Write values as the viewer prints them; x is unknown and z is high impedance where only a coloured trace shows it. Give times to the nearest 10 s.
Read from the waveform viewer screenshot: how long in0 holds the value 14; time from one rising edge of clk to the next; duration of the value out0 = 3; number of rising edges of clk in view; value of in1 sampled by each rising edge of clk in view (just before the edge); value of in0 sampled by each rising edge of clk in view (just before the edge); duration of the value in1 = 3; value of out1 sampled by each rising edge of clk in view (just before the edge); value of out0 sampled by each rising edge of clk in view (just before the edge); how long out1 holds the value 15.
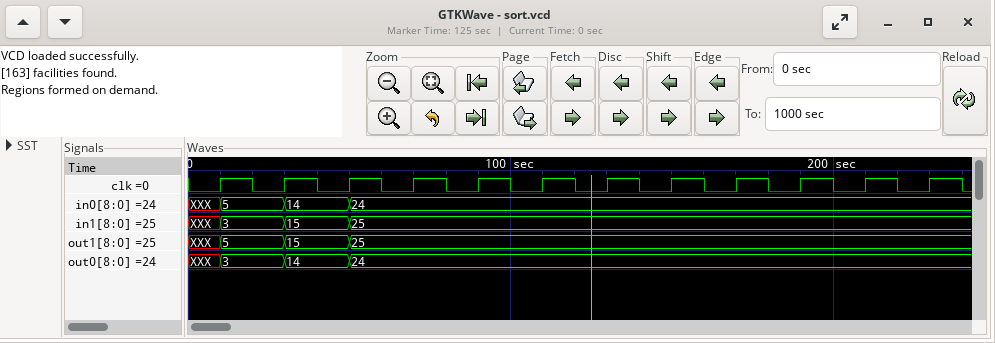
20 s
20 s
20 s
12
XXX, 3, 15, 25, 25, 25, 25, 25, 25, 25, 25, 25
XXX, 5, 14, 24, 24, 24, 24, 24, 24, 24, 24, 24
20 s
XXX, 5, 15, 25, 25, 25, 25, 25, 25, 25, 25, 25
XXX, 3, 14, 24, 24, 24, 24, 24, 24, 24, 24, 24
20 s
